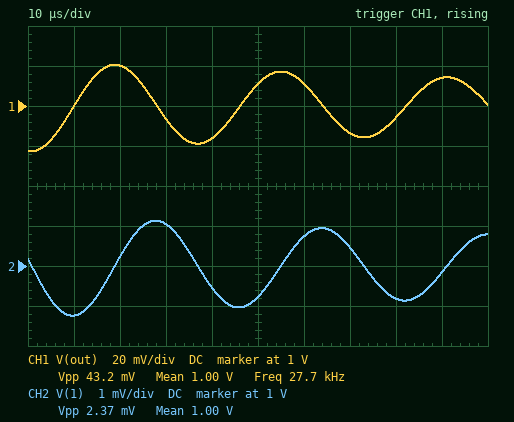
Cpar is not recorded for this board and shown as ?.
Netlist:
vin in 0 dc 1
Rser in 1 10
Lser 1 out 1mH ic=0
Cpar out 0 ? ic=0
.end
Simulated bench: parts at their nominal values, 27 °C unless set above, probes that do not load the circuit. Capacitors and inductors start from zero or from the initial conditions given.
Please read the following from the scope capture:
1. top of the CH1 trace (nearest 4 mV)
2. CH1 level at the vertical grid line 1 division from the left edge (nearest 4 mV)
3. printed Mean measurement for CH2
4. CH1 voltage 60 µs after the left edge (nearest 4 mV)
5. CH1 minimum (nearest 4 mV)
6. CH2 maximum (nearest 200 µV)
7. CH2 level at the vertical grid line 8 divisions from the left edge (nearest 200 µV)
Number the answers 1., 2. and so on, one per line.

1. 1.020 V
2. 1.000 V
3. 1.00 V
4. 1.012 V
5. 976 mV
6. 1.0012 V
7. 999.2 mV
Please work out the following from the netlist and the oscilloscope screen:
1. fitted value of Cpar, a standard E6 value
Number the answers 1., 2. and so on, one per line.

1. 33 nF
